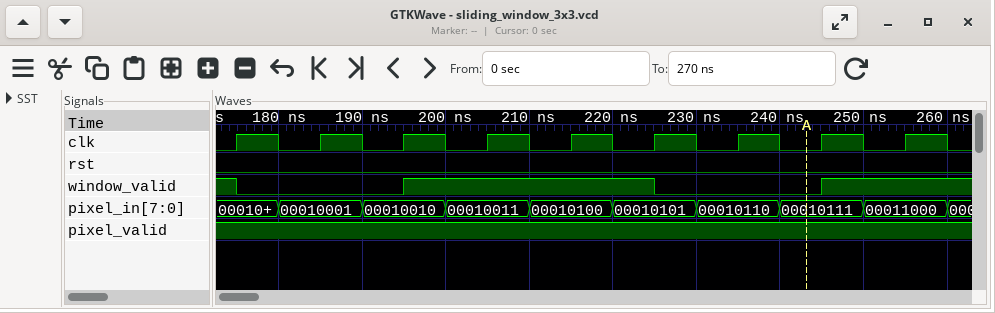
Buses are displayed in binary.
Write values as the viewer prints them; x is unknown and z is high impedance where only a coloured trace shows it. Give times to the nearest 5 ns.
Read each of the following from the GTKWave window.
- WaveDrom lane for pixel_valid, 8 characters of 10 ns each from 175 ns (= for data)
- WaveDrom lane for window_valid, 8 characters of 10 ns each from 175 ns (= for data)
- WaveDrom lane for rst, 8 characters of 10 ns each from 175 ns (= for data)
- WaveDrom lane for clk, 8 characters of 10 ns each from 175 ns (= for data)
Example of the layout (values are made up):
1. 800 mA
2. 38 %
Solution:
1. {name: 'pixel_valid', wave: '1.......'}
2. {name: 'window_valid', wave: '0.1..0.1'}
3. {name: 'rst', wave: '0.......'}
4. {name: 'clk', wave: 'p.......'}
